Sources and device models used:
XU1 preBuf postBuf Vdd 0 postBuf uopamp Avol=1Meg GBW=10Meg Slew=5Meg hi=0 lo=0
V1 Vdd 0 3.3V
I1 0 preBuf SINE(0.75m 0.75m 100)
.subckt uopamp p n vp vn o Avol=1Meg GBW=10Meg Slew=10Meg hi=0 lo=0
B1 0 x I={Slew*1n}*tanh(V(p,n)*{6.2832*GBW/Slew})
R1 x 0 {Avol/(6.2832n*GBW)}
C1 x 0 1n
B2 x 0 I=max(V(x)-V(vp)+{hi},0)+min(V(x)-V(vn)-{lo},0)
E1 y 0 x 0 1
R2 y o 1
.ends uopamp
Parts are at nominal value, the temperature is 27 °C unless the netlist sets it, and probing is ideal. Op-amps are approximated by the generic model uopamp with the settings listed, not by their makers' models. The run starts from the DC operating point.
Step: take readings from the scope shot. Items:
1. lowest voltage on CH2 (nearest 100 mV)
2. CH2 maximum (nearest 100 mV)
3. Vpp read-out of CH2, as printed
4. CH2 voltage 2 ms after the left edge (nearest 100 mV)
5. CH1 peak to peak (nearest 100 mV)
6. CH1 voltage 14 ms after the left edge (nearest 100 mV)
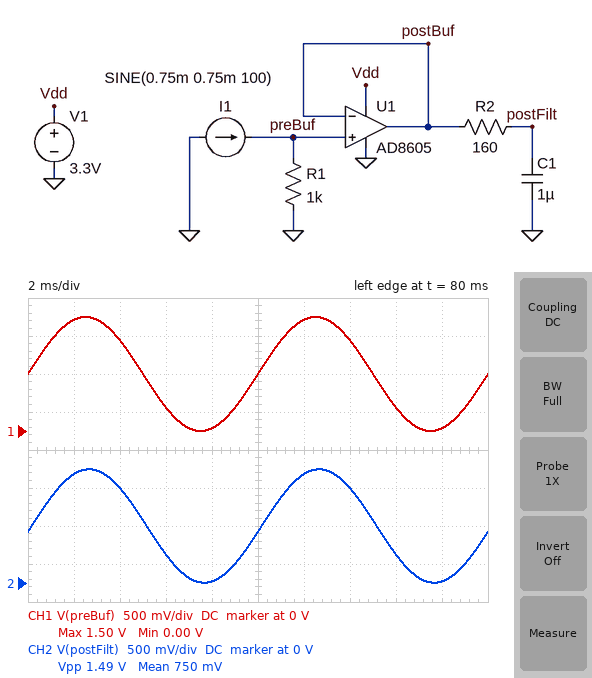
0 V
1.5 V
1.49 V
1.4 V
1.5 V
1.2 V
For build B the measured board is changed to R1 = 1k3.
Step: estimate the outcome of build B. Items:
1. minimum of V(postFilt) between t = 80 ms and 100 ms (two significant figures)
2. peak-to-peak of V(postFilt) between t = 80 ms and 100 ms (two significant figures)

4.9 mV
1.9 V
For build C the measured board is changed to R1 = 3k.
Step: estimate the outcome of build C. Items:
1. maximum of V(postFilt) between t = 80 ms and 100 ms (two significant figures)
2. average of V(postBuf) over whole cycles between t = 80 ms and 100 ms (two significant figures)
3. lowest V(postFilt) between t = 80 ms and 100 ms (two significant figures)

3.3 V
2.0 V
11 mV
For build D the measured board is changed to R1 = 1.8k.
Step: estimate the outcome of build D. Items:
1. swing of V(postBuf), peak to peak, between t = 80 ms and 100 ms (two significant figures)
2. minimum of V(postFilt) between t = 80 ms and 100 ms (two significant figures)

2.7 V
6.8 mV
